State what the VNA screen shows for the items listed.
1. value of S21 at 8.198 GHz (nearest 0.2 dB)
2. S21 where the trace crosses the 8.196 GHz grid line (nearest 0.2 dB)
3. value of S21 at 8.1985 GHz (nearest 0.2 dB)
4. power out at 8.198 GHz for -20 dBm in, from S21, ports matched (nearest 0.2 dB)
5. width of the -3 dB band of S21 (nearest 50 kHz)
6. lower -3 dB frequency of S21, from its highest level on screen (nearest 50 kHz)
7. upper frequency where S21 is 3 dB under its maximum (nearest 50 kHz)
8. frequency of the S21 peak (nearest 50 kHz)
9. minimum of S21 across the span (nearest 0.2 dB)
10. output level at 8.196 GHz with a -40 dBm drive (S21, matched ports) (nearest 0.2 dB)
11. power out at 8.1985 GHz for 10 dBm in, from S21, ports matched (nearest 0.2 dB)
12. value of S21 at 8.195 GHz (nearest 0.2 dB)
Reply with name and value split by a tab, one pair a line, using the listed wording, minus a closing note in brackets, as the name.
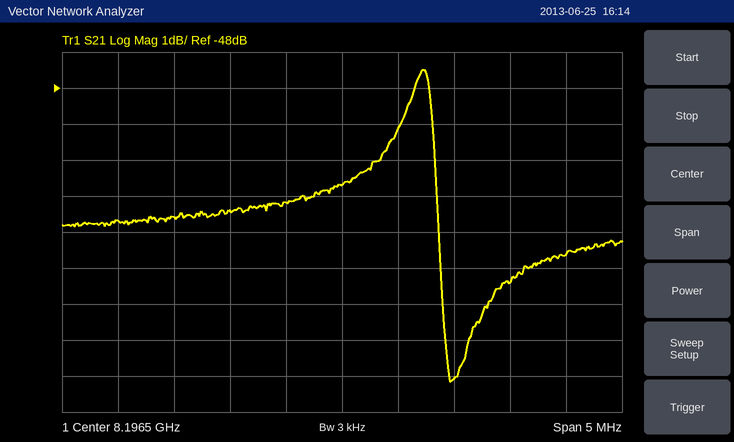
value of S21 at 8.198 GHz	-53.4 dB
S21 where the trace crosses the 8.196 GHz grid line	-51.2 dB
value of S21 at 8.1985 GHz	-52.6 dB
power out at 8.198 GHz for -20 dBm in, from S21, ports matched	-73.4 dBm
width of the -3 dB band of S21	750 kHz
lower -3 dB frequency of S21, from its highest level on screen	8.19660 GHz
upper frequency where S21 is 3 dB under its maximum	8.19735 GHz
frequency of the S21 peak	8.19720 GHz
minimum of S21 across the span	-56.2 dB
output level at 8.196 GHz with a -40 dBm drive (S21, matched ports)	-91.2 dBm
power out at 8.1985 GHz for 10 dBm in, from S21, ports matched	-42.6 dBm
value of S21 at 8.195 GHz	-51.6 dB
